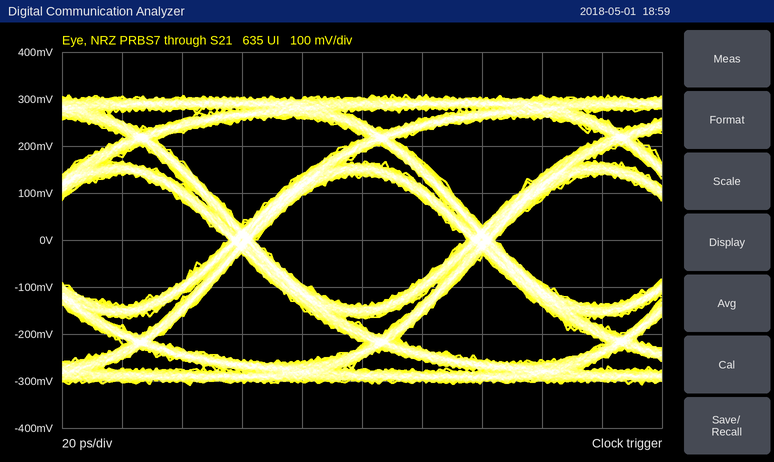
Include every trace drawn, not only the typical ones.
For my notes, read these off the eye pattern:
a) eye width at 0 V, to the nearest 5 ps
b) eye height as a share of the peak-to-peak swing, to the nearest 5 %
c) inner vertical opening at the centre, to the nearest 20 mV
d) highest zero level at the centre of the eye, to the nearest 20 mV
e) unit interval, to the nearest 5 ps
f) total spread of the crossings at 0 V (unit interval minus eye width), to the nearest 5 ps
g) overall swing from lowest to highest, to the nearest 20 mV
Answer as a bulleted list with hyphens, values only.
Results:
- 70 ps
- 45 %
- 280 mV
- -140 mV
- 80 ps
- 10 ps
- 620 mV
